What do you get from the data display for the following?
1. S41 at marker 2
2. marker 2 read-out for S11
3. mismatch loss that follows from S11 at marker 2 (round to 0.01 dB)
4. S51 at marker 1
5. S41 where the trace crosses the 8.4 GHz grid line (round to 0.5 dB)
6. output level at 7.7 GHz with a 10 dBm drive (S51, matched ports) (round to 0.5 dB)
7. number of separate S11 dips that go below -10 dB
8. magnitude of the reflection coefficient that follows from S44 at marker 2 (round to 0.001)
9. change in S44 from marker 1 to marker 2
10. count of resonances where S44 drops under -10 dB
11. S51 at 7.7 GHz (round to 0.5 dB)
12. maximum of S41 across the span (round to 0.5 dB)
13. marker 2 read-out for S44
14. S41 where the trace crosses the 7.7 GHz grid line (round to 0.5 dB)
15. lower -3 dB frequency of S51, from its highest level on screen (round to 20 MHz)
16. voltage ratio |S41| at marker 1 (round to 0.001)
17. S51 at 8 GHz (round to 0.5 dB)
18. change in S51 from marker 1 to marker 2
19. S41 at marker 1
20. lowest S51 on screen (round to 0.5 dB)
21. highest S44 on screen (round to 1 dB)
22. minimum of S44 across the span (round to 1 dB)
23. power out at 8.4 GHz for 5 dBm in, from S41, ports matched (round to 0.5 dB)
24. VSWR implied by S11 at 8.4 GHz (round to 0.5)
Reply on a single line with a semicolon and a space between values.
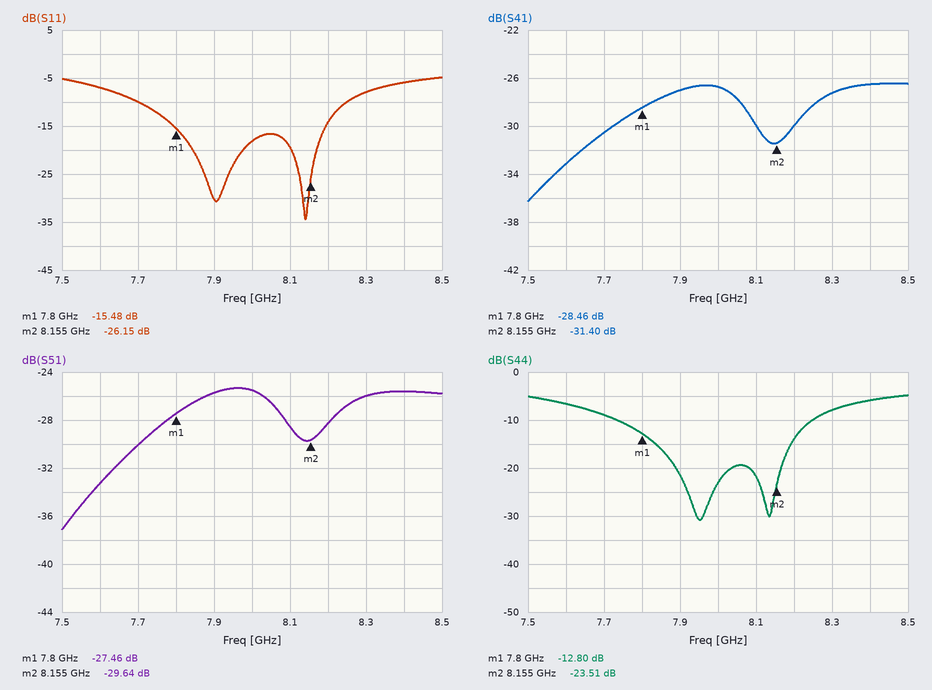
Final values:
-31.40 dB; -26.15 dB; 0.01 dB; -27.46 dB; -26.5 dB; -20.0 dBm; 2; 0.067; -10.71 dB; 2; -30.0 dB; -26.5 dB; -23.51 dB; -30.5 dB; 7.76 GHz; 0.038; -25.5 dB; -2.18 dB; -28.46 dB; -37.0 dB; -5 dB; -31 dB; -21.5 dBm; 3.0
